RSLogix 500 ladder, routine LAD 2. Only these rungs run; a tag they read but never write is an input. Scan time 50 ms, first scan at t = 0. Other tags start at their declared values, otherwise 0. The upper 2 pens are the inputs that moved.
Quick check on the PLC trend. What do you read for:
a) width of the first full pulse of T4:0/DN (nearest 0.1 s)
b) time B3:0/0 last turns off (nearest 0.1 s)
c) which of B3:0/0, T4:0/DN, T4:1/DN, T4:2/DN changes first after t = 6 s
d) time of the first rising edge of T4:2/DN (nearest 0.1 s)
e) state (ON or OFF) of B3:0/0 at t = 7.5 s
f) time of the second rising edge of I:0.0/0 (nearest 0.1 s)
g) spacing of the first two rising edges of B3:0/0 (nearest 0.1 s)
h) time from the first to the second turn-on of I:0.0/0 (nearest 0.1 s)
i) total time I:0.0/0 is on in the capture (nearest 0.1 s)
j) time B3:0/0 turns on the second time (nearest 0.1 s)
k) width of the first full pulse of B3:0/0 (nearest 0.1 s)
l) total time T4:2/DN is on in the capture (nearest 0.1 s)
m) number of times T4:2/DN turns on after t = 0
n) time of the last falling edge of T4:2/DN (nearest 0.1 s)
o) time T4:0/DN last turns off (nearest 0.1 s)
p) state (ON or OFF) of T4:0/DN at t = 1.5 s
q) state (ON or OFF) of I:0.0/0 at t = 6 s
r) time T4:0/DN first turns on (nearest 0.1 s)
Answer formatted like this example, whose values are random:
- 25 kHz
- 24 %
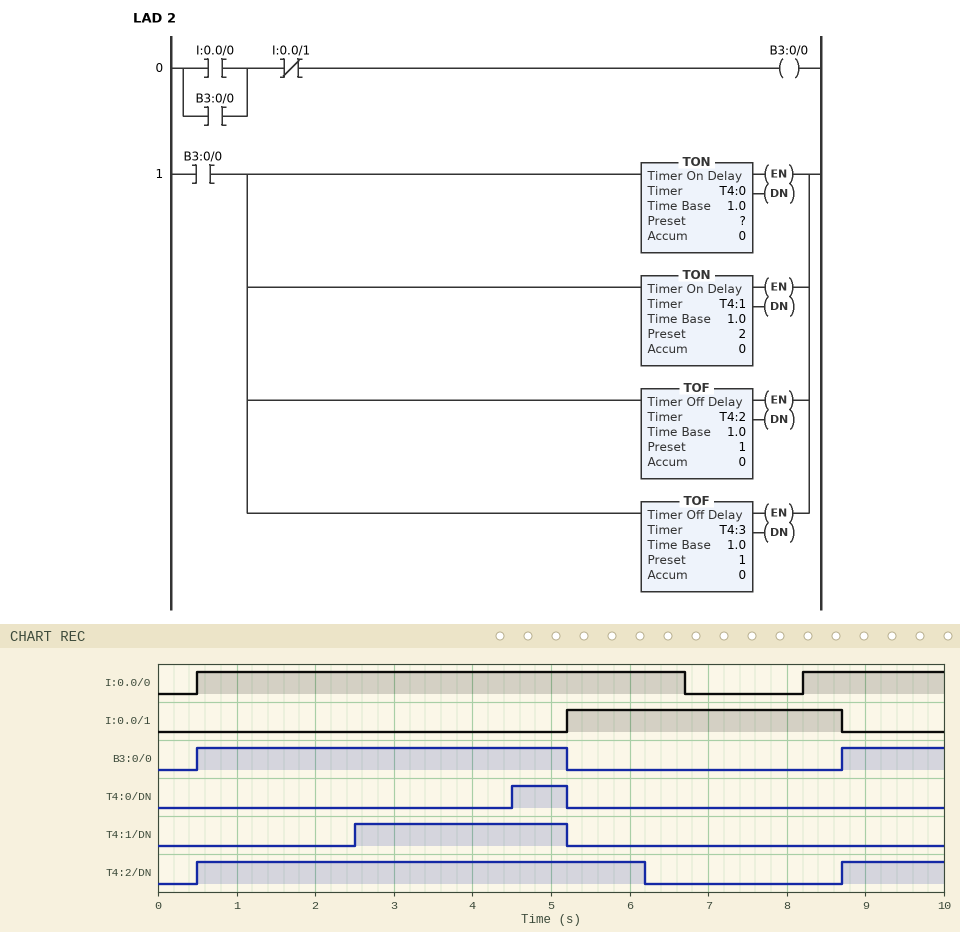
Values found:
- 0.7 s
- 5.2 s
- T4:2/DN
- 0.5 s
- OFF
- 8.2 s
- 8.2 s
- 7.7 s
- 8.0 s
- 8.7 s
- 4.7 s
- 7.0 s
- 2
- 6.2 s
- 5.2 s
- OFF
- ON
- 4.5 s
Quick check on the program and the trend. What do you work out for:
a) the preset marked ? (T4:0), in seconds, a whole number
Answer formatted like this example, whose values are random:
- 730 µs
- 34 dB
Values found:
- 4 s
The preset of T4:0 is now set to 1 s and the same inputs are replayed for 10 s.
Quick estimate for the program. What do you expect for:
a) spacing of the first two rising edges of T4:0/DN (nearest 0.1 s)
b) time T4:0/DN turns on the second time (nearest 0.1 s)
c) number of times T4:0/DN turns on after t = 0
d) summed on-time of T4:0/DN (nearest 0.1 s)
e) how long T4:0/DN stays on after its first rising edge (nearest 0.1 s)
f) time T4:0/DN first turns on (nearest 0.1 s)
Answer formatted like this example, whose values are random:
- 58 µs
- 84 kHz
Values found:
- 8.2 s
- 9.7 s
- 2
- 4.0 s
- 3.7 s
- 1.5 s
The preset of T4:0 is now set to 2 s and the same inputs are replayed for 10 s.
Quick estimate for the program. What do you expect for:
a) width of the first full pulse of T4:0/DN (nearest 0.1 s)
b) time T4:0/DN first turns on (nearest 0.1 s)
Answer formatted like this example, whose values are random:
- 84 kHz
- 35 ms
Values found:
- 2.7 s
- 2.5 s
